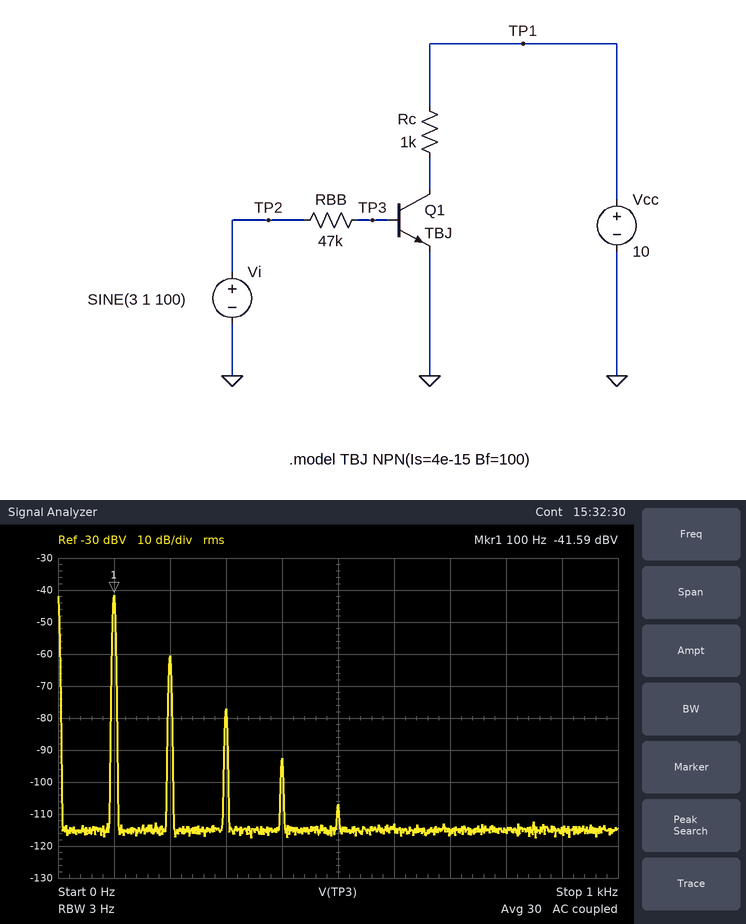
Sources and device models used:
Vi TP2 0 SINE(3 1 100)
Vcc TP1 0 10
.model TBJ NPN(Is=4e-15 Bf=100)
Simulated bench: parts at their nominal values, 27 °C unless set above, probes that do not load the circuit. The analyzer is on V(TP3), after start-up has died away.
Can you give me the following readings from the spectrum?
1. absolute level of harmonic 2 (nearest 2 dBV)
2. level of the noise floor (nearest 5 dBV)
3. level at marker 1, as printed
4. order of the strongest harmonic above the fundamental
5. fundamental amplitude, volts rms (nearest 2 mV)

-60 dBV
-115 dBV
-41.59 dBV
2
8 mV
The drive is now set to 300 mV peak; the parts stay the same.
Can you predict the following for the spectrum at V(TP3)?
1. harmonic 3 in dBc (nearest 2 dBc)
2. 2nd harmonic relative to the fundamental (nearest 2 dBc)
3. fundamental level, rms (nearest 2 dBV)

-58 dBc
-30 dBc
-52 dBV
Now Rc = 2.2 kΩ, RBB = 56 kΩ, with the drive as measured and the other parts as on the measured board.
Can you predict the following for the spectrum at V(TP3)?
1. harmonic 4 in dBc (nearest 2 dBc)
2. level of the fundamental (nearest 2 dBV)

-30 dBc
-44 dBV
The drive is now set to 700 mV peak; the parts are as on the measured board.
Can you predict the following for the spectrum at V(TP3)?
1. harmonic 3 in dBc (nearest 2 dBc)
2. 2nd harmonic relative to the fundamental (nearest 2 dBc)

-42 dBc
-22 dBc
